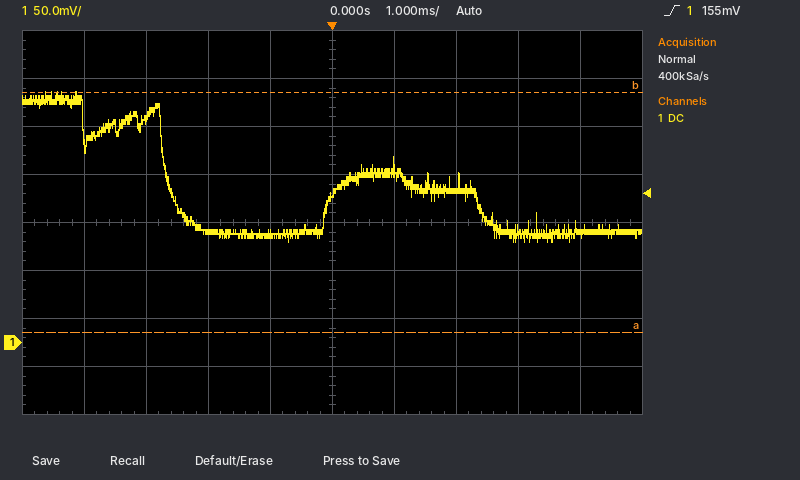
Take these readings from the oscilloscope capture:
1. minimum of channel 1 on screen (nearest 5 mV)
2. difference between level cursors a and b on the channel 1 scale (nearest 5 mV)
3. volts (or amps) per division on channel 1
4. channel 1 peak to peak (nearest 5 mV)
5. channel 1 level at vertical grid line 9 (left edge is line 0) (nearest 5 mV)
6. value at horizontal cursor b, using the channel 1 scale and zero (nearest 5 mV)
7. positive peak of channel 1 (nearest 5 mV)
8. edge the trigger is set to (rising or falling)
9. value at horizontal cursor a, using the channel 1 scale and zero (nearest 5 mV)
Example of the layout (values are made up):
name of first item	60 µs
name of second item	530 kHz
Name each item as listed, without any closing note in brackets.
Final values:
minimum of channel 1 on screen	105 mV
difference between level cursors a and b on the channel 1 scale	250 mV
volts (or amps) per division on channel 1	50 mV
channel 1 peak to peak	155 mV
channel 1 level at vertical grid line 9 (left edge is line 0)	115 mV
value at horizontal cursor b, using the channel 1 scale and zero	260 mV
positive peak of channel 1	260 mV
edge the trigger is set to	rising
value at horizontal cursor a, using the channel 1 scale and zero	10 mV
